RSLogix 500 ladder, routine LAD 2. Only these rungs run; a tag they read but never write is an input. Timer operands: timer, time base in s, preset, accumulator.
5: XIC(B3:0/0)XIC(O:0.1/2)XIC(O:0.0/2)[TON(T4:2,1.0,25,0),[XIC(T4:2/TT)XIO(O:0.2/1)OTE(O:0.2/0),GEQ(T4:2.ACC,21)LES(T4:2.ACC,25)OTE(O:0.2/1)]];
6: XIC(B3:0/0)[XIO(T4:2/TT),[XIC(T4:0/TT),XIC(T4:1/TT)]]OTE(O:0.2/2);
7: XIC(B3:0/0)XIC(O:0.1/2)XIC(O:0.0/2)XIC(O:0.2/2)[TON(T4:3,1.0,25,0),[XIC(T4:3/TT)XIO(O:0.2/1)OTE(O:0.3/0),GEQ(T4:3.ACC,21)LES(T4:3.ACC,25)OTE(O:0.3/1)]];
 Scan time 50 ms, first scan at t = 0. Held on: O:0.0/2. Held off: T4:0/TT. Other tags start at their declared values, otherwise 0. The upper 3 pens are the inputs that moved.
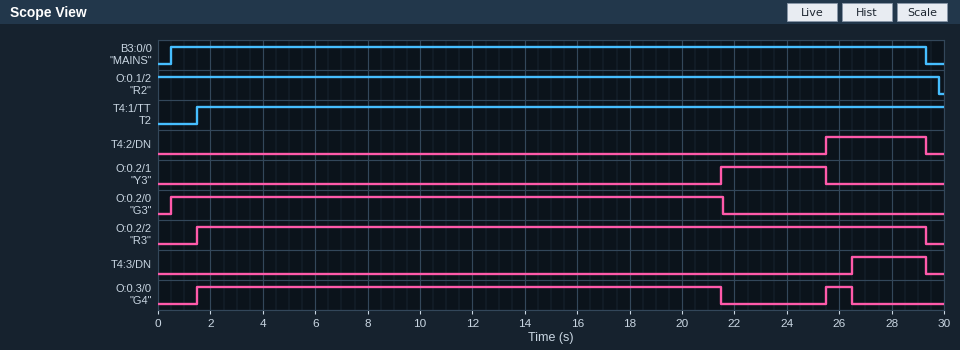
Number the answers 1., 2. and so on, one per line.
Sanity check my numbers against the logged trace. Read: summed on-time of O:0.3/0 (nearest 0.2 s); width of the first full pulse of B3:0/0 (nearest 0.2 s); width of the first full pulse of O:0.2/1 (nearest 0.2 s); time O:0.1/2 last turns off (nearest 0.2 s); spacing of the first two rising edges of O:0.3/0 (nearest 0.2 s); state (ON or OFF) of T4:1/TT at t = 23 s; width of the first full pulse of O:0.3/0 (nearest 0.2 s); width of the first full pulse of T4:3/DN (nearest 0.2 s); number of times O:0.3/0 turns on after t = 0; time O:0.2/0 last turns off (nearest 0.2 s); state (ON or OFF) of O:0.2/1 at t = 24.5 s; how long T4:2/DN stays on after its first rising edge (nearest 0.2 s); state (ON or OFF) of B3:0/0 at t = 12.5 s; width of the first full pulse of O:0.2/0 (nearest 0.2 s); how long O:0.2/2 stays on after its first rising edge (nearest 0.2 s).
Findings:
1. 21.0 s
2. 28.8 s
3. 4.0 s
4. 29.8 s
5. 24.0 s
6. ON
7. 20.0 s
8. 2.8 s
9. 2
10. 21.6 s
11. ON
12. 3.8 s
13. ON
14. 21.0 s
15. 27.8 s
